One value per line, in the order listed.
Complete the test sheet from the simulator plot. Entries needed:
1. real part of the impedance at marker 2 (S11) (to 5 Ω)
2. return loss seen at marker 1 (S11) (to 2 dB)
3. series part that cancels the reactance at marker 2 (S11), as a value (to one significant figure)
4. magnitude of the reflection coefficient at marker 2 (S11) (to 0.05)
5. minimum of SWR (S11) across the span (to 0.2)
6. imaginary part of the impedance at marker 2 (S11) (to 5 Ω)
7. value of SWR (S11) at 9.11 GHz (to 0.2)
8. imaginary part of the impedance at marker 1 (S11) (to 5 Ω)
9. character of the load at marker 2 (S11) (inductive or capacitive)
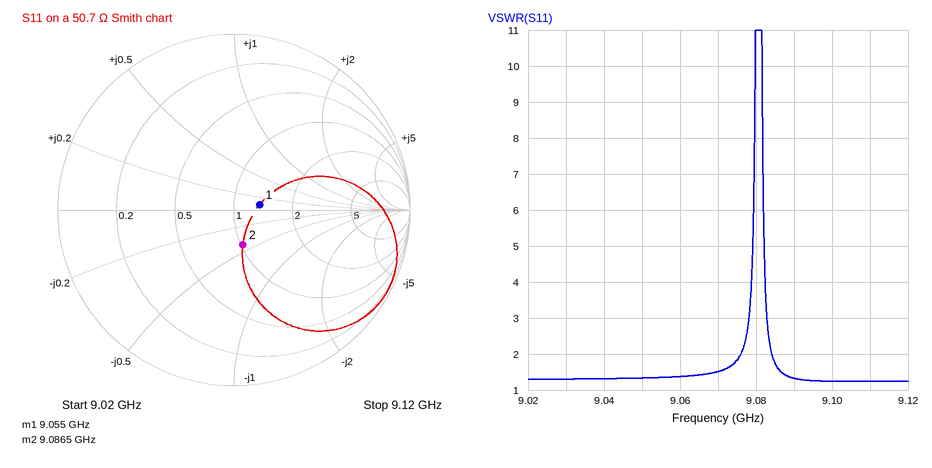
50 Ω
16 dB
400 pH
0.20
1.2
-20 Ω
1.2
+5 Ω
capacitive
